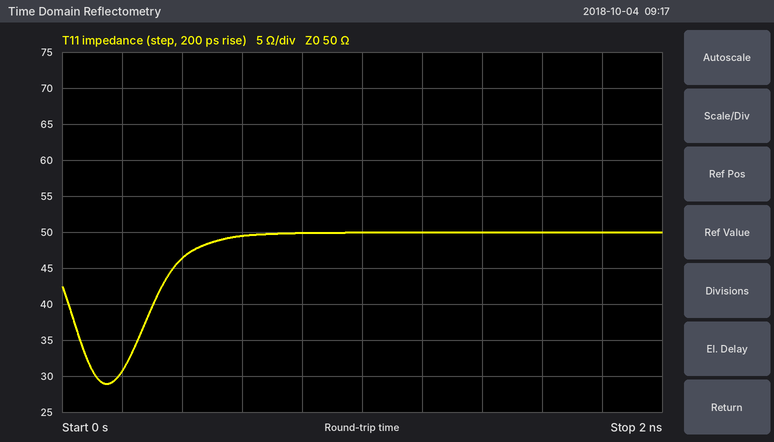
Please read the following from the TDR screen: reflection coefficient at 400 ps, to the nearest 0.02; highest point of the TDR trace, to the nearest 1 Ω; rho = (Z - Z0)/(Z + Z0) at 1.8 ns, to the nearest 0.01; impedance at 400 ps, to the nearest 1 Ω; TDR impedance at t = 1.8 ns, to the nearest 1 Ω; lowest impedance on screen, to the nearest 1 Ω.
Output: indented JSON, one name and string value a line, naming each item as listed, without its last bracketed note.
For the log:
{
  "reflection coefficient at 400 ps, to the nearest 0.02": "-0.04",
  "highest point of the TDR trace, to the nearest 1 Ω": "50 Ω",
  "rho = (Z - Z0)/(Z + Z0) at 1.8 ns, to the nearest 0.01": "0.00",
  "impedance at 400 ps, to the nearest 1 Ω": "46 Ω",
  "TDR impedance at t = 1.8 ns, to the nearest 1 Ω": "50 Ω",
  "lowest impedance on screen, to the nearest 1 Ω": "29 Ω"
}
